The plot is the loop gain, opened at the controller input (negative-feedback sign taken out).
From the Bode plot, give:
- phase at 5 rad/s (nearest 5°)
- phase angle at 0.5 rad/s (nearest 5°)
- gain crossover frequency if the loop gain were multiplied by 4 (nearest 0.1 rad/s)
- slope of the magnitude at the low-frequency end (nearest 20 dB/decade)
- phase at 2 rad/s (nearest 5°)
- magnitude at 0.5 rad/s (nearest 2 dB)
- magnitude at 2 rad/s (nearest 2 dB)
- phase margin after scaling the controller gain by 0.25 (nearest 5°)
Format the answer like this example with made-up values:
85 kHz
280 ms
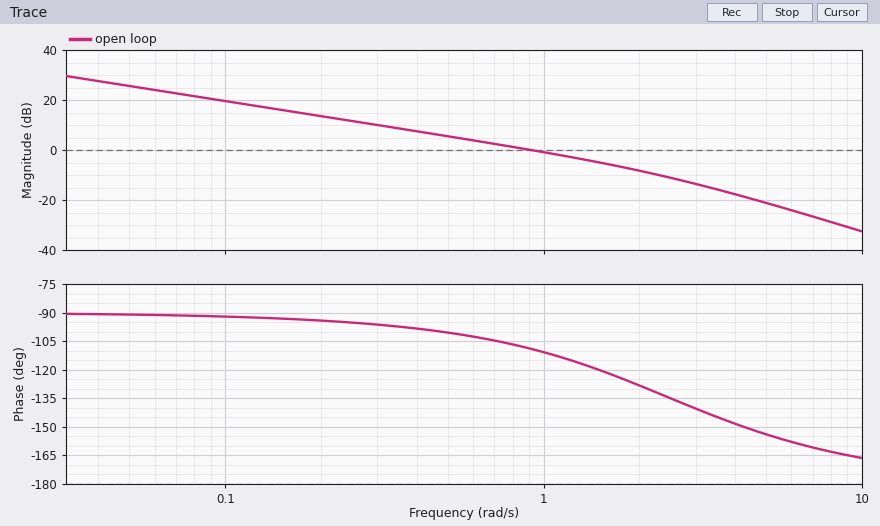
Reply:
-155°
-100°
2.7 rad/s
-20 dB/decade
-130°
6 dB
-8 dB
85°
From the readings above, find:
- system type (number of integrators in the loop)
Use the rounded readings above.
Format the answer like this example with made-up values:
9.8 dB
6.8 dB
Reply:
1
